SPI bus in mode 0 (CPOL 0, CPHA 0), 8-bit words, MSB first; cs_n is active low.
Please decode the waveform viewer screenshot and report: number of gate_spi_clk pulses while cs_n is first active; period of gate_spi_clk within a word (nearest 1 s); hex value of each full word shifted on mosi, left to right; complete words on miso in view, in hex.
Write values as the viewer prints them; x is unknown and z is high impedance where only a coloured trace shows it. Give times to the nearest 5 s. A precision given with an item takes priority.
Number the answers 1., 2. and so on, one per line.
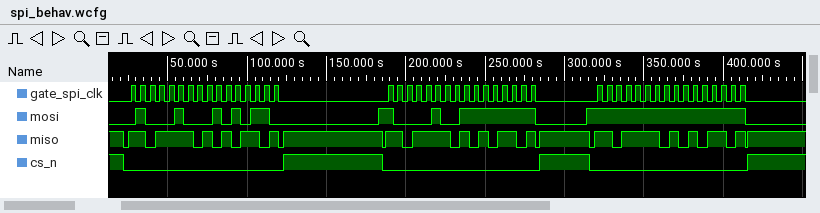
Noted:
1. 16
2. 6 s
3. 44, 56, 84, FF, FF, FF
4. DE, AD, DE, AD, DE, AD
